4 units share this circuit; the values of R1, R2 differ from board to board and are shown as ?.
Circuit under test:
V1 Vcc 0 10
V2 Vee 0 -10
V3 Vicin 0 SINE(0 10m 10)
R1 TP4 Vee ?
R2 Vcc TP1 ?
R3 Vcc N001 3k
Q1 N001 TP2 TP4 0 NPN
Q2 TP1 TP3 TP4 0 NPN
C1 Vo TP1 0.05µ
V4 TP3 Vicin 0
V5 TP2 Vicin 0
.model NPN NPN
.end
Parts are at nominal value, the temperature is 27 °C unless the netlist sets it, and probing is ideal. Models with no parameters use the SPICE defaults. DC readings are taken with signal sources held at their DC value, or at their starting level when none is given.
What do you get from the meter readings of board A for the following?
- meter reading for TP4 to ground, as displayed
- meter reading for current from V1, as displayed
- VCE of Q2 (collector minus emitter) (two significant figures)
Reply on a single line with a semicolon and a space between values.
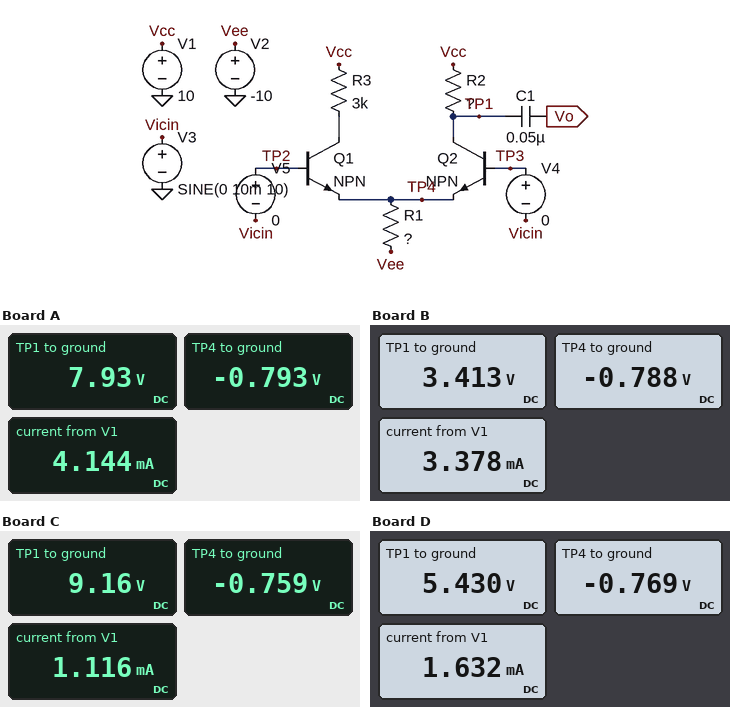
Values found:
-0.793 V; 4.144 mA; 8.7 V
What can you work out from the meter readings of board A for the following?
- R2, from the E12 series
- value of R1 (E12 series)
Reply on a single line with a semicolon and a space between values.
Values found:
1 kΩ; 2.2 kΩ
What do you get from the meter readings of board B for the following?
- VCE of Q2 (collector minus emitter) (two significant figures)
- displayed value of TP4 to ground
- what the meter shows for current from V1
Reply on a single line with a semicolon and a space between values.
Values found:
4.2 V; -0.788 V; 3.378 mA
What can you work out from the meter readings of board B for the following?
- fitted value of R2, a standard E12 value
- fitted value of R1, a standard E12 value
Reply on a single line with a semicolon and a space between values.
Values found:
3.9 kΩ; 2.7 kΩ
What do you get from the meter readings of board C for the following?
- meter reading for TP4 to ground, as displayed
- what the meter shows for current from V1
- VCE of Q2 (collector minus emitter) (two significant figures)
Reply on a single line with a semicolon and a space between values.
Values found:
-0.759 V; 1.116 mA; 9.9 V
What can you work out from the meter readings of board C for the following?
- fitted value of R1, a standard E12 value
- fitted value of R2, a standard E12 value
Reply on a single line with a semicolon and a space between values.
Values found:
8.2 kΩ; 1.5 kΩ
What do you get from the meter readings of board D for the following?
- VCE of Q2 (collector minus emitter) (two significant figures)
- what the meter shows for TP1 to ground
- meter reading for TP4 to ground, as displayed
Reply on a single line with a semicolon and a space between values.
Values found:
6.2 V; 5.430 V; -0.769 V
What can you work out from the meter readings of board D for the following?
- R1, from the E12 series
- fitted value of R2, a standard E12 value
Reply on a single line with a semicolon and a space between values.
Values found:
5.6 kΩ; 5.6 kΩ
